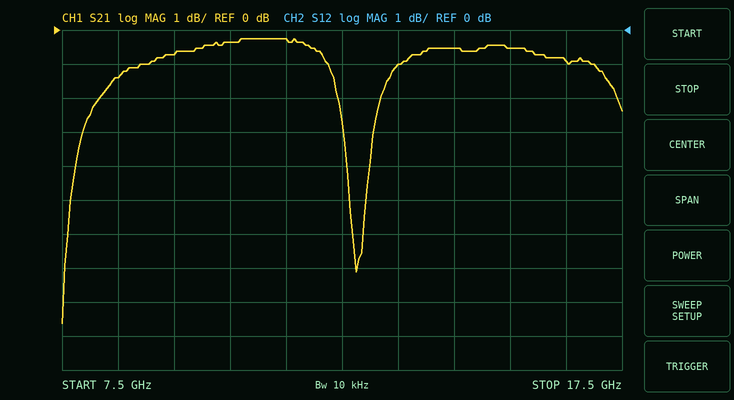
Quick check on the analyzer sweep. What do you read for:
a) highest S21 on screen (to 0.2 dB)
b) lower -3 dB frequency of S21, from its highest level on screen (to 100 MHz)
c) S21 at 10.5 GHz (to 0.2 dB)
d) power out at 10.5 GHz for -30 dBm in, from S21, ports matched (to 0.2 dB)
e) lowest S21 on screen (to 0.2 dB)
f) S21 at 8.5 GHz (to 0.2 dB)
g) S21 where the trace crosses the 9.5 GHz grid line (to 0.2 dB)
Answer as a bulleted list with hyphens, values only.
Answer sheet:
- -0.2 dB
- 7.8 GHz
- -0.4 dB
- -30.4 dBm
- -8.6 dB
- -1.4 dB
- -0.8 dB
